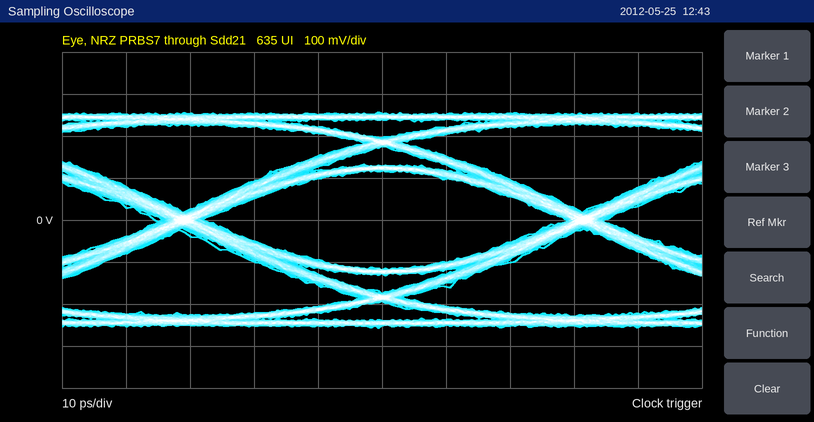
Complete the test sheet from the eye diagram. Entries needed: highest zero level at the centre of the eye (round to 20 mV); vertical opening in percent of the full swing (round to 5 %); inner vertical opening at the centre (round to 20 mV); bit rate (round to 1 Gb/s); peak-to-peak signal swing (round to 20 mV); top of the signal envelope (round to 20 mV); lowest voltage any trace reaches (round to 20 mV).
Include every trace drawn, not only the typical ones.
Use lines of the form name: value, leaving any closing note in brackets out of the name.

highest zero level at the centre of the eye: -120 mV
vertical opening in percent of the full swing: 45 %
inner vertical opening at the centre: 240 mV
bit rate: 16 Gb/s
peak-to-peak signal swing: 520 mV
top of the signal envelope: 260 mV
lowest voltage any trace reaches: -260 mV
